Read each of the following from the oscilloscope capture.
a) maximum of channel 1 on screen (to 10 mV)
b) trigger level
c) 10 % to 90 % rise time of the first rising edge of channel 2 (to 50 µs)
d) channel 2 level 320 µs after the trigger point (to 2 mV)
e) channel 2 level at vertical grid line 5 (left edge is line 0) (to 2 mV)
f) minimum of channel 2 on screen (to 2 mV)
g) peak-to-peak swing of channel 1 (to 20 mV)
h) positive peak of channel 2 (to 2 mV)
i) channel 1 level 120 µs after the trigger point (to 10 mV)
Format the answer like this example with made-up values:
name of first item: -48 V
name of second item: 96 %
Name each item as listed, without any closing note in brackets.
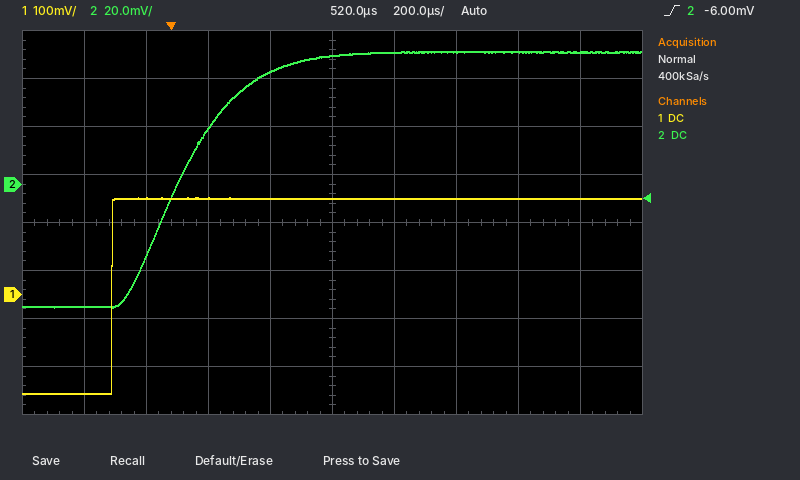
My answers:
maximum of channel 1 on screen: 200 mV
trigger level: -6.00 mV
10 % to 90 % rise time of the first rising edge of channel 2: 400 µs
channel 2 level 320 µs after the trigger point: 46 mV
channel 2 level at vertical grid line 5 (left edge is line 0): 54 mV
minimum of channel 2 on screen: -52 mV
peak-to-peak swing of channel 1: 400 mV
positive peak of channel 2: 56 mV
channel 1 level 120 µs after the trigger point: 200 mV
